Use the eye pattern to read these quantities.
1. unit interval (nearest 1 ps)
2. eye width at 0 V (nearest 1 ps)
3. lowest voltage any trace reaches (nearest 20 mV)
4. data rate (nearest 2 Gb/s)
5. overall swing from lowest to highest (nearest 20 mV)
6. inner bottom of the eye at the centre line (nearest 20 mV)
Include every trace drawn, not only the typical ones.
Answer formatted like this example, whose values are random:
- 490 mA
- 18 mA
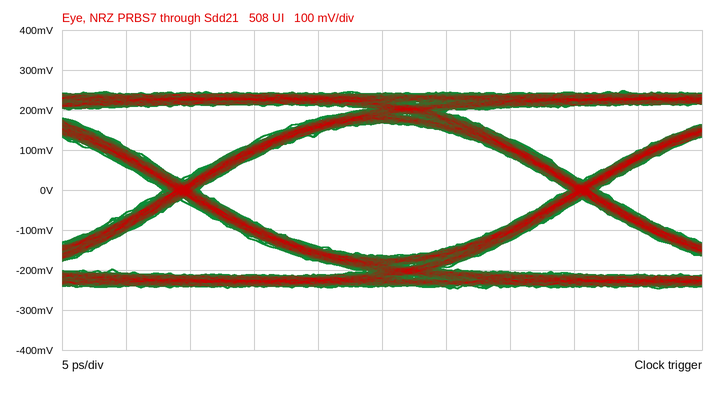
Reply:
- 31 ps
- 29 ps
- -240 mV
- 32 Gb/s
- 500 mV
- -160 mV
